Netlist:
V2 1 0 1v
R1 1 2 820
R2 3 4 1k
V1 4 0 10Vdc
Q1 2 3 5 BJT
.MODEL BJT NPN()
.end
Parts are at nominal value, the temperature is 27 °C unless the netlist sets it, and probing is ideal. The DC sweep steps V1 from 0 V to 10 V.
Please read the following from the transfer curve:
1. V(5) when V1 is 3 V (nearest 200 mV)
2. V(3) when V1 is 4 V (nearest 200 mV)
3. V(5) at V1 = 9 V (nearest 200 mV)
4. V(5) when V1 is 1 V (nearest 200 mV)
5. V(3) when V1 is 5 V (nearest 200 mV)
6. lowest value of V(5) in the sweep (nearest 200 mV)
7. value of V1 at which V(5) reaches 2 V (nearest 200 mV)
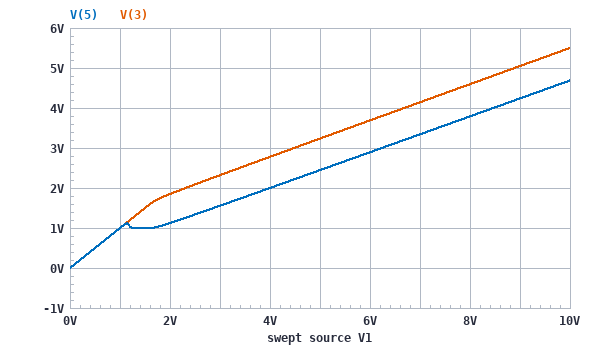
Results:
1.6 V
2.8 V
4.2 V
1.0 V
3.2 V
0 V
4.0 V
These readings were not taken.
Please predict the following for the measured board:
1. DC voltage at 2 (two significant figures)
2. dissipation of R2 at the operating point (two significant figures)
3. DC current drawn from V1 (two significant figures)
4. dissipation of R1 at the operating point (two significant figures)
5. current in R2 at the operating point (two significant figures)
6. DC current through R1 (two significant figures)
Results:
4.7 V
20 mW
4.5 mA
17 mW
4.5 mA
4.5 mA
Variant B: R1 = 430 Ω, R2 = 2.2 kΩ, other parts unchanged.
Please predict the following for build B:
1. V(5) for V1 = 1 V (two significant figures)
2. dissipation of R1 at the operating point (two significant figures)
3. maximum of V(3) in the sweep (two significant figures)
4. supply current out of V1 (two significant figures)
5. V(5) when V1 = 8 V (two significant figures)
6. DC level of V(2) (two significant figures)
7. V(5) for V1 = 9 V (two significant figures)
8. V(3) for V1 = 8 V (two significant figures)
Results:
1.0 V
4.2 mW
3.1 V
3.1 mA
2.0 V
2.3 V
2.2 V
2.8 V
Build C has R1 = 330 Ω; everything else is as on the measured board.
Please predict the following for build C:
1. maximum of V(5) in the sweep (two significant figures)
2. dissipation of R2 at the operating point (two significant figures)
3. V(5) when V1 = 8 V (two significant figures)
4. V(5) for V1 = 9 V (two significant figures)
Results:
3.0 V
38 mW
2.5 V
2.8 V
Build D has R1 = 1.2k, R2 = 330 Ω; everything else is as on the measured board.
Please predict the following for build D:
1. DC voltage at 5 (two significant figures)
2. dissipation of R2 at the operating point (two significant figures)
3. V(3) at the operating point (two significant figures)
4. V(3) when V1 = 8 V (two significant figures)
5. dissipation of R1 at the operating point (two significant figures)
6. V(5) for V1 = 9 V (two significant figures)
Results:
7.4 V
9.4 mW
8.2 V
6.7 V
34 mW
6.6 V
